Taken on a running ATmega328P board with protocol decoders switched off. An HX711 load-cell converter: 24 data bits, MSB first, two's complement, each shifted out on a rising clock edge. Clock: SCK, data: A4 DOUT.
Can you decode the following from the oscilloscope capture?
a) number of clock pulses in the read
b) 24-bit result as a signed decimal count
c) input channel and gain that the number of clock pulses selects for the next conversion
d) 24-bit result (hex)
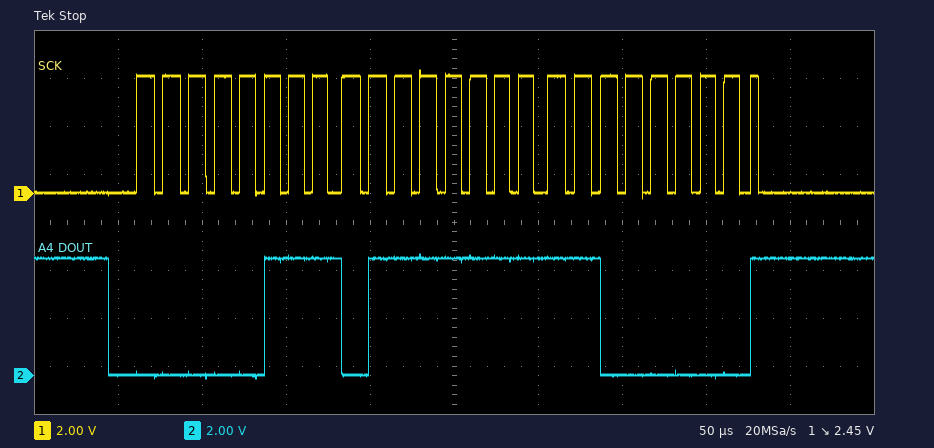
25
491456
channel A, gain 128
0x077FC0
